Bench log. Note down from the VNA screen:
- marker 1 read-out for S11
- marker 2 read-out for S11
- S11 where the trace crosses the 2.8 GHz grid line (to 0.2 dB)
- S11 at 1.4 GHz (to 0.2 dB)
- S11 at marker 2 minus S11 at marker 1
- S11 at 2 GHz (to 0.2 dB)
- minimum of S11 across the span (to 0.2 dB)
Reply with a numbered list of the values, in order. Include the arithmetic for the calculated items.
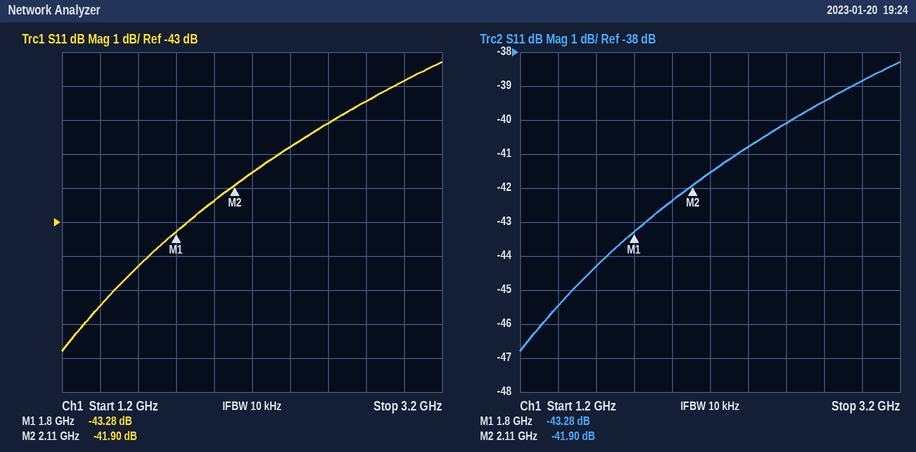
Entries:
1. -43.28 dB
2. -41.90 dB
3. -39.4 dB
4. -45.4 dB
5. -41.9 − (-43.28) = 1.38 dB
6. -42.4 dB
7. -46.8 dB
